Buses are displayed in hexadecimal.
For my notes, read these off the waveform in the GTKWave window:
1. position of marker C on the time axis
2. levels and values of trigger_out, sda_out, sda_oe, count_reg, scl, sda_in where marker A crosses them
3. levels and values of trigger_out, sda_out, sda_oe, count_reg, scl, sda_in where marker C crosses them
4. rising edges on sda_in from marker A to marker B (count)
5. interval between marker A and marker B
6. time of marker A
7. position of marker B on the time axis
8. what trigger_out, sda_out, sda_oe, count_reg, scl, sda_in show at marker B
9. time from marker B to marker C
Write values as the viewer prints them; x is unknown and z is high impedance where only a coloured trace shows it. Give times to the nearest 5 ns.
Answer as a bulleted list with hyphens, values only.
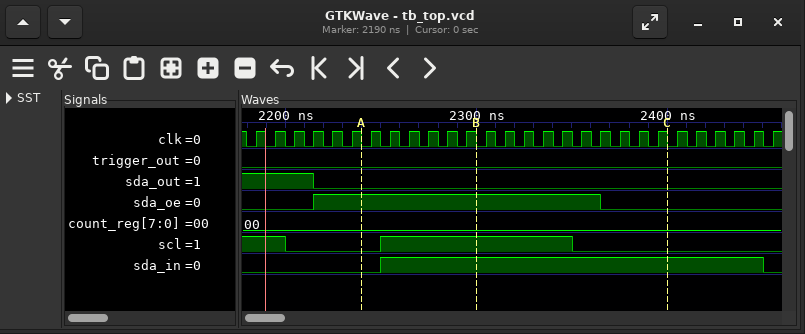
- 2400 ns
- trigger_out=0, sda_out=0, sda_oe=1, count_reg=00, scl=0, sda_in=0
- trigger_out=0, sda_out=0, sda_oe=0, count_reg=00, scl=0, sda_in=1
- 1
- 60 ns
- 2240 ns
- 2300 ns
- trigger_out=0, sda_out=0, sda_oe=1, count_reg=00, scl=1, sda_in=1
- 100 ns
